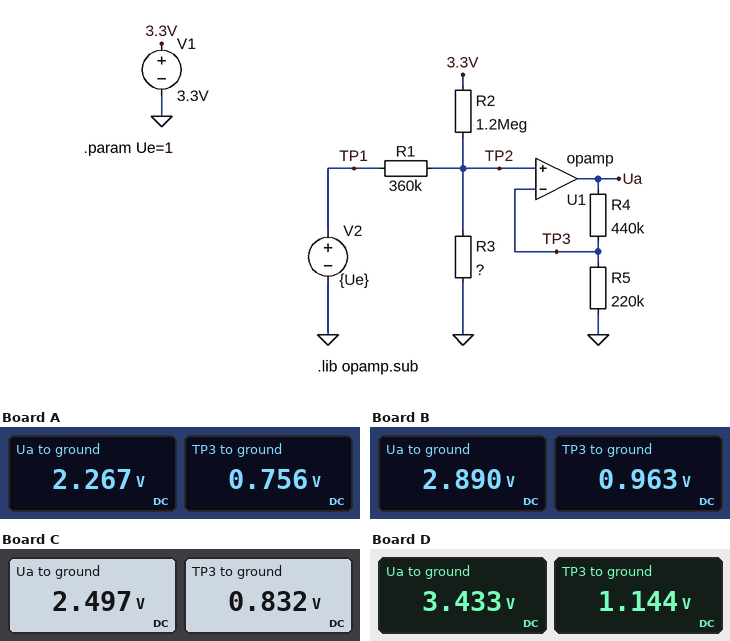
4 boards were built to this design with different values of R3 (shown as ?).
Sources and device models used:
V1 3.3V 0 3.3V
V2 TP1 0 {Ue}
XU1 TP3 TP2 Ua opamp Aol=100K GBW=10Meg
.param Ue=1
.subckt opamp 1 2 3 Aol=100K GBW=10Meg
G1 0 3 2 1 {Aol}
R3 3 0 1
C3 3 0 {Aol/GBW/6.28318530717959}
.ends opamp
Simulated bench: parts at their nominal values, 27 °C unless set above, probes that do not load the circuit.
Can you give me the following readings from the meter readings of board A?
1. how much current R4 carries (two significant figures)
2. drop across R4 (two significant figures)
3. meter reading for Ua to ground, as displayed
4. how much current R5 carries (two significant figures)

3.4 µA
1.5 V
2.267 V
3.4 µA
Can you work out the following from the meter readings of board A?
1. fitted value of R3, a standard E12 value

270 kΩ
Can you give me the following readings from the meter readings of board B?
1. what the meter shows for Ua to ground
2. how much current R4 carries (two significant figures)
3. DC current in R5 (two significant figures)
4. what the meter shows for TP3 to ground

2.890 V
4.4 µA
4.4 µA
0.963 V
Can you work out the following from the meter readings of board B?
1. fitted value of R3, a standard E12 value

470 kΩ
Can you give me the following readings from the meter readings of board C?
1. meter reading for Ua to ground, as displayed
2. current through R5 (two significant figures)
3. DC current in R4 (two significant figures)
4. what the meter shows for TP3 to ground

2.497 V
3.8 µA
3.8 µA
0.832 V
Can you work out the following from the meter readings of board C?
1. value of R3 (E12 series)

330 kΩ
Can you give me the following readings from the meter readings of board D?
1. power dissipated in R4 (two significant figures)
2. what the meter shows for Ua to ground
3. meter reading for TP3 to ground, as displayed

12 µW
3.433 V
1.144 V
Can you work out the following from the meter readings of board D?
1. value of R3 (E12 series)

820 kΩ
